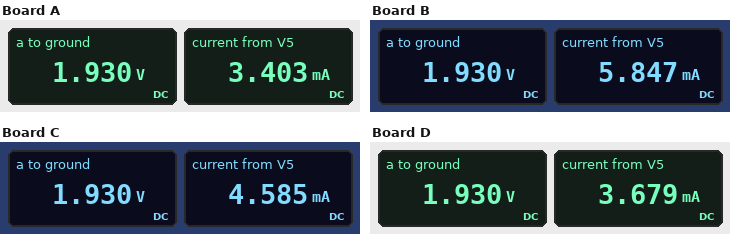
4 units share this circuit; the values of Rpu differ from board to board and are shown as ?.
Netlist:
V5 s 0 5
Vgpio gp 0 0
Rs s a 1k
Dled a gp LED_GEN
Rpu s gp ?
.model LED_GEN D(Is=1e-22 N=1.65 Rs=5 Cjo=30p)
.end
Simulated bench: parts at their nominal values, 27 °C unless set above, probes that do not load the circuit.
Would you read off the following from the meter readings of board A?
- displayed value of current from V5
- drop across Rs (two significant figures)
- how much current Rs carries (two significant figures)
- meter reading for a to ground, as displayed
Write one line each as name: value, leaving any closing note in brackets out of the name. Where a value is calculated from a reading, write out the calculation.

displayed value of current from V5: 3.403 mA
drop across Rs: 5 V - 1.93 V = 3.1 V
how much current Rs carries: (5 V - 1.93 V) / 1 kΩ = 3.1 mA
meter reading for a to ground, as displayed: 1.930 V
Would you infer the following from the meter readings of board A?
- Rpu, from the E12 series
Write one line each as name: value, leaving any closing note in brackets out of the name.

Rpu, from the E12 series: 15 kΩ
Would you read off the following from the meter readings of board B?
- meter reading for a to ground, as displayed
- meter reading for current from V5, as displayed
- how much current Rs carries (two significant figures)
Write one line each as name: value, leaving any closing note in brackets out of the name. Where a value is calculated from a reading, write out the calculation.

meter reading for a to ground, as displayed: 1.930 V
meter reading for current from V5, as displayed: 5.847 mA
how much current Rs carries: (5 V - 1.93 V) / 1 kΩ = 3.1 mA
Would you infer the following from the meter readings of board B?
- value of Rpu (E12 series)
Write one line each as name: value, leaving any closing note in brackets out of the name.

value of Rpu: 1.8 kΩ
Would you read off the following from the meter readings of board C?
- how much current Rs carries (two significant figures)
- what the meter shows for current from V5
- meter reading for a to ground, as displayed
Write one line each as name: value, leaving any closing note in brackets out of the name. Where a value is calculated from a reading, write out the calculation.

how much current Rs carries: (5 V - 1.93 V) / 1 kΩ = 3.1 mA
what the meter shows for current from V5: 4.585 mA
meter reading for a to ground, as displayed: 1.930 V
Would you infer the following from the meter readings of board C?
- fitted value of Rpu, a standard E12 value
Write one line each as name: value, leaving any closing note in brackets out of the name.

fitted value of Rpu, a standard E12 value: 3.3 kΩ
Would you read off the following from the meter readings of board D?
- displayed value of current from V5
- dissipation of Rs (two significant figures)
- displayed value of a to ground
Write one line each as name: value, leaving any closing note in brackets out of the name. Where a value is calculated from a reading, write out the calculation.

displayed value of current from V5: 3.679 mA
dissipation of Rs: (5 V - 1.93 V)^2 / 1 kΩ = 9.4 mW
displayed value of a to ground: 1.930 V
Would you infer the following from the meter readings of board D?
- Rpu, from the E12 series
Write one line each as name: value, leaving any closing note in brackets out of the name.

Rpu, from the E12 series: 8.2 kΩ
